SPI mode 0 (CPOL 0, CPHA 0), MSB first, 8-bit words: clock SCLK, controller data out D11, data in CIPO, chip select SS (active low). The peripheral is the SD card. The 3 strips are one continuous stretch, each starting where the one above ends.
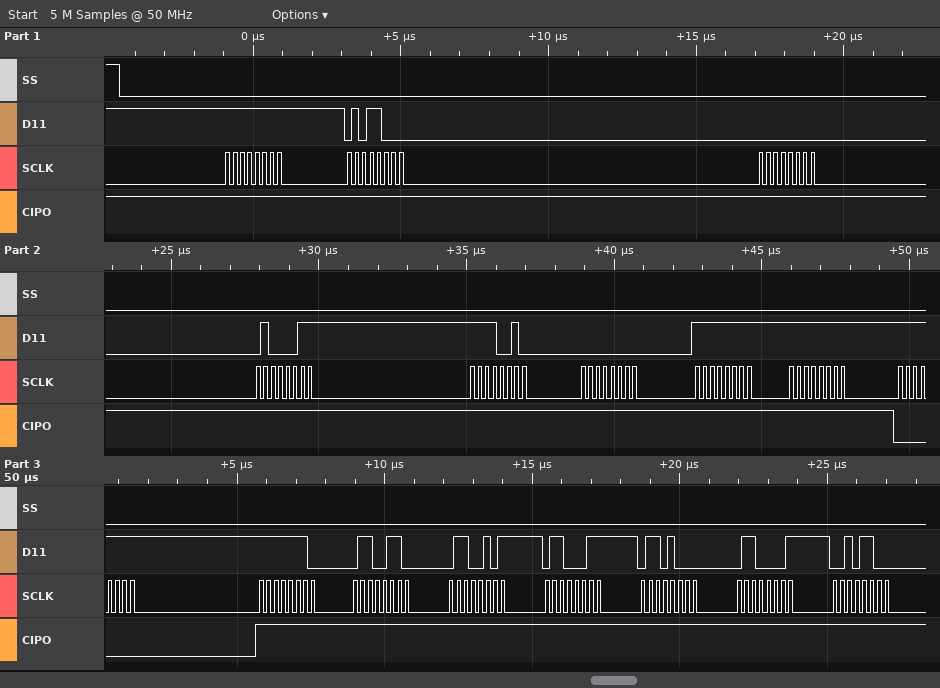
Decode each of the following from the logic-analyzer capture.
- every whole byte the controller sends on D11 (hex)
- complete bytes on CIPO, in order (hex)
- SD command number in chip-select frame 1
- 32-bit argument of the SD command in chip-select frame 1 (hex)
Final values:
0xFF 0x58 0x00 0x43 0xF2 0x00 0xFF 0xFF 0xFF 0xFE 0x66 0x65 0x63 0x68 0x61 0x2C
0xFF 0xFF 0xFF 0xFF 0xFF 0xFF 0xFF 0xFF 0x00 0xFF 0xFF 0xFF 0xFF 0xFF 0xFF 0xFF
CMD24
0x0043F200
